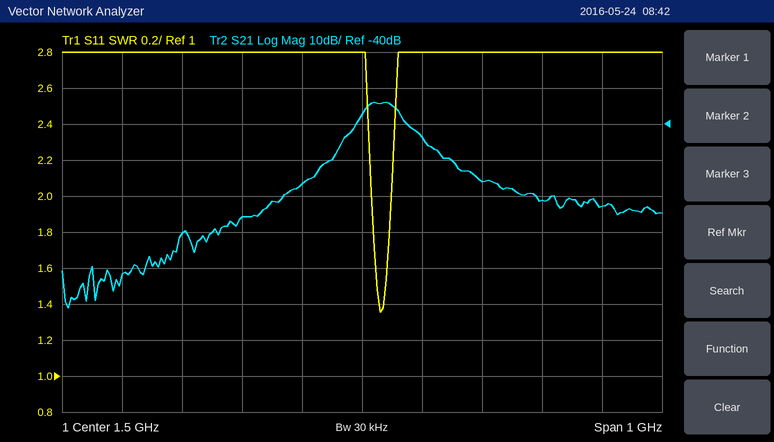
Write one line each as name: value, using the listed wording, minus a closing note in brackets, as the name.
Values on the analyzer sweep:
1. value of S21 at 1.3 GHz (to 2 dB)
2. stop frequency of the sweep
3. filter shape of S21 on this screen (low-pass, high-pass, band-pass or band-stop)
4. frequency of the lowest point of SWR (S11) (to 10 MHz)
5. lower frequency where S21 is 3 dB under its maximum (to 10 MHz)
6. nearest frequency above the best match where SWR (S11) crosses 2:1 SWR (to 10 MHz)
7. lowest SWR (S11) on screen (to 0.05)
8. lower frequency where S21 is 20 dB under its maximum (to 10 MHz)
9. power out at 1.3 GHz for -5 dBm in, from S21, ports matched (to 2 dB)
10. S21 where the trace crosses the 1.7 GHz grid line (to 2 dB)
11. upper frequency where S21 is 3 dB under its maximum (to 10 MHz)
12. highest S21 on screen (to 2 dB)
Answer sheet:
value of S21 at 1.3 GHz: -66 dB
stop frequency of the sweep: 2 GHz
filter shape of S21 on this screen: band-pass
frequency of the lowest point of SWR (S11): 1.53 GHz
lower frequency where S21 is 3 dB under its maximum: 1.50 GHz
nearest frequency above the best match where SWR (S11) crosses 2:1 SWR: 1.55 GHz
lowest SWR (S11) on screen: 1.35
lower frequency where S21 is 20 dB under its maximum: 1.42 GHz
power out at 1.3 GHz for -5 dBm in, from S21, ports matched: -70 dBm
S21 where the trace crosses the 1.7 GHz grid line: -56 dB
upper frequency where S21 is 3 dB under its maximum: 1.56 GHz
highest S21 on screen: -34 dB
